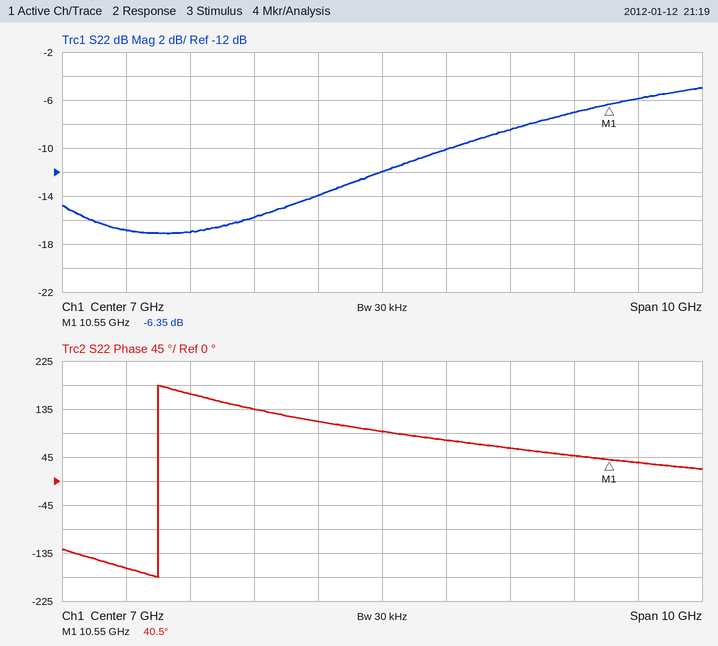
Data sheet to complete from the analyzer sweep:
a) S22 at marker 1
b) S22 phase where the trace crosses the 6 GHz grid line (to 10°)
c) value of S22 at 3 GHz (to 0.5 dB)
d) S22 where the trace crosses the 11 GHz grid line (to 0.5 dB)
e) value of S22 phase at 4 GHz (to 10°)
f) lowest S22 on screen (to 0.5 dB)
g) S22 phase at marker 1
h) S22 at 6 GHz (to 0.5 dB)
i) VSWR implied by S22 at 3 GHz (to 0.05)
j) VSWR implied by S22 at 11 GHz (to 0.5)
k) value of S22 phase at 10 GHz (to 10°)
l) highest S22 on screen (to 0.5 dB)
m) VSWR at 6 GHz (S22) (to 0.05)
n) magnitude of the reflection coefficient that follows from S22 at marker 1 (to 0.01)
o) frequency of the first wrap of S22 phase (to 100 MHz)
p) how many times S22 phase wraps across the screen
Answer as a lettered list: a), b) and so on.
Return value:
a) -6.35 dB
b) 110°
c) -17.0 dB
d) -6.0 dB
e) 160°
f) -17.0 dB
g) 40.5°
h) -14.0 dB
i) 1.35
j) 3.0
k) 50°
l) -5.0 dB
m) 1.50
n) 0.48
o) 3.5 GHz
p) 1
